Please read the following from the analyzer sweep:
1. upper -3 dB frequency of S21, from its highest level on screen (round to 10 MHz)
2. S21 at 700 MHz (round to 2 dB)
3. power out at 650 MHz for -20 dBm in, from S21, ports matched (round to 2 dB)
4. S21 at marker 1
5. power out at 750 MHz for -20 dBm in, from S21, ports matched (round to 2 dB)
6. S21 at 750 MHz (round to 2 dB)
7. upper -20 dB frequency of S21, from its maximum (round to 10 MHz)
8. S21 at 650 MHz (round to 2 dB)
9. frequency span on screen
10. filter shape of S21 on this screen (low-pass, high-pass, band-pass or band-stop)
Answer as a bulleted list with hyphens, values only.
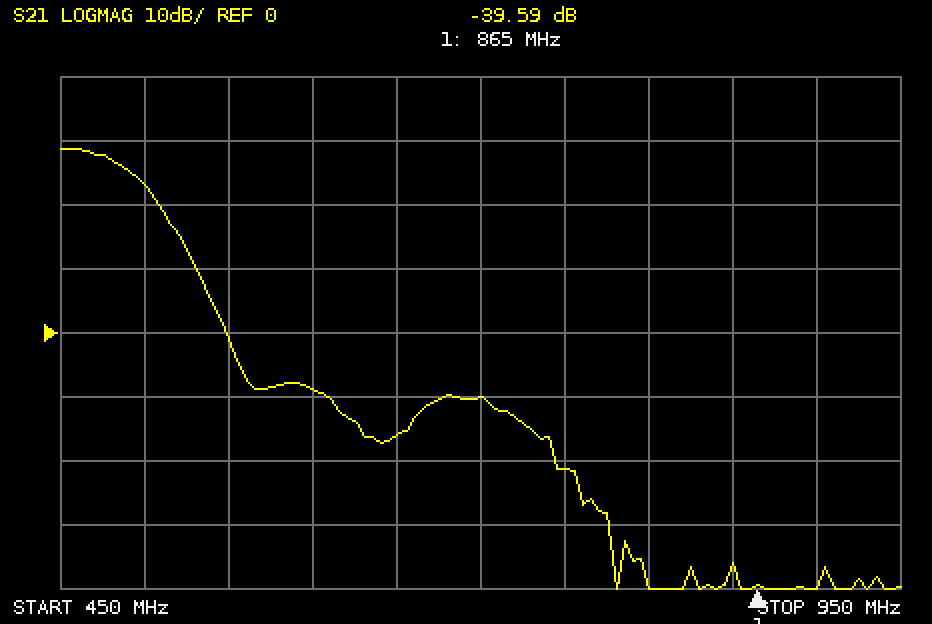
- 490 MHz
- -10 dB
- -36 dBm
- -39.59 dB
- -42 dBm
- -22 dB
- 530 MHz
- -16 dB
- 500 MHz
- low-pass
